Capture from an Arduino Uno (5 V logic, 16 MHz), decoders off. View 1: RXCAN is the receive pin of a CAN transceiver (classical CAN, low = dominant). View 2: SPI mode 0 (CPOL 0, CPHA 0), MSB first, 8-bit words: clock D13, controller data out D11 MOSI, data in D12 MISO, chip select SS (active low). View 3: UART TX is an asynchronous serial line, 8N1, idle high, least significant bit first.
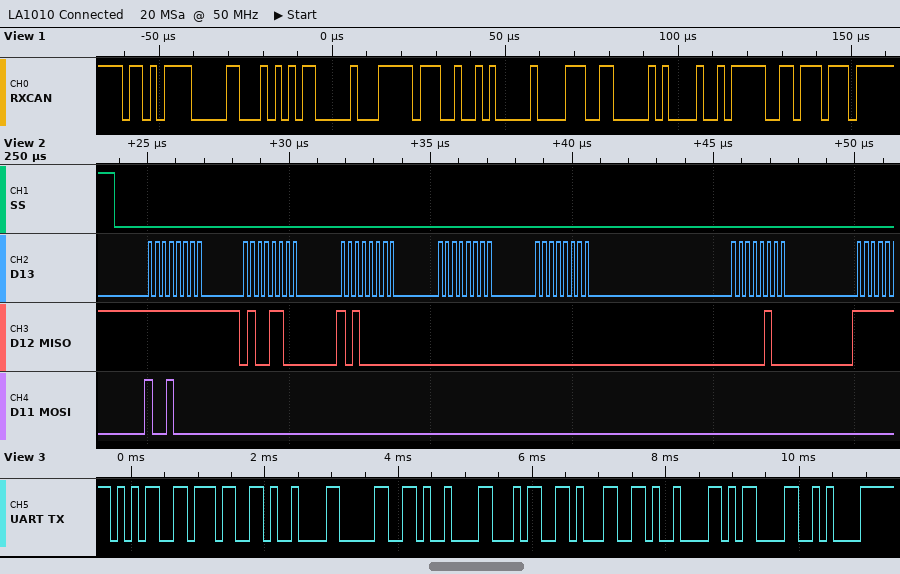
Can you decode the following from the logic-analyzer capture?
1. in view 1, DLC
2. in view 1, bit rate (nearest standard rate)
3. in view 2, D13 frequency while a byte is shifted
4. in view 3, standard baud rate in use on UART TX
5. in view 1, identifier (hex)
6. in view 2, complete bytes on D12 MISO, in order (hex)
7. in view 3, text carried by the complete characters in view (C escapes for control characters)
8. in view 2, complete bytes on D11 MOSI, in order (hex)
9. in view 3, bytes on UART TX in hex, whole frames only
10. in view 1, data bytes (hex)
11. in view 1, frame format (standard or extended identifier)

8
500 kbit/s
4 MHz
9600 baud
0x6BC
FF 4C A0 00 00 04
"57\t0\t41\t\r\n"
90 00 00 00 00 00
35 37 09 30 09 34 31 09 0D 0A
AB 00 FF 25 00 73 02 12
standard
